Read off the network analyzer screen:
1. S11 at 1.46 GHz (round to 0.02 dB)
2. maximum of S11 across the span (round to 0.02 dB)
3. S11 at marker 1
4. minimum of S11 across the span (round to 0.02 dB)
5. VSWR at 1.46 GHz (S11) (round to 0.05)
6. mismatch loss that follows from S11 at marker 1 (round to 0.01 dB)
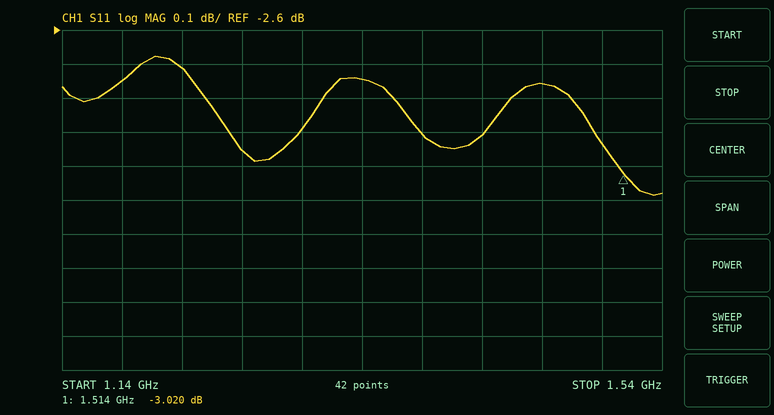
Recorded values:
-2.76 dB
-2.68 dB
-3.020 dB
-3.08 dB
6.35
3.00 dB
